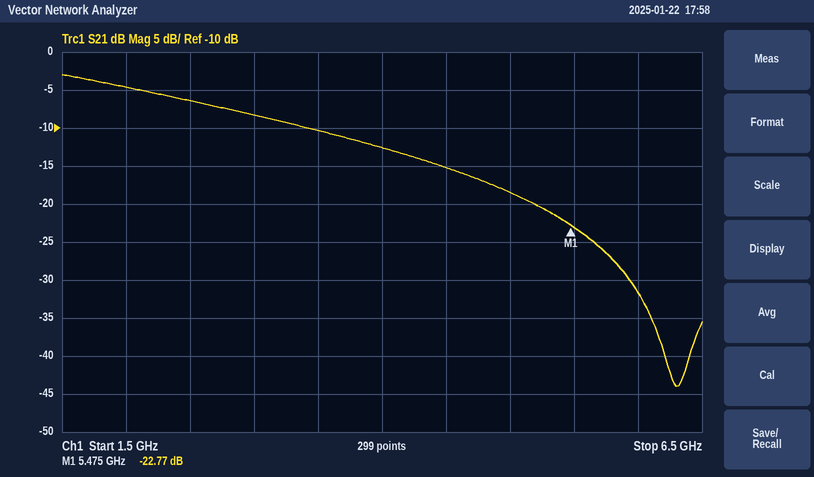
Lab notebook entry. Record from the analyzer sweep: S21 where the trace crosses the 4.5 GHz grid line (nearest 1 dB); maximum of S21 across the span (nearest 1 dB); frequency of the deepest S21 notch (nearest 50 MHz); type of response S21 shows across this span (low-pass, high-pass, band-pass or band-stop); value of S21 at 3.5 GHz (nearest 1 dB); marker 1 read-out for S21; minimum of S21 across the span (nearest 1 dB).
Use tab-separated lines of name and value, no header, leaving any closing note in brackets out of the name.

S21 where the trace crosses the 4.5 GHz grid line	-15 dB
maximum of S21 across the span	-3 dB
frequency of the deepest S21 notch	6.30 GHz
type of response S21 shows across this span	low-pass
value of S21 at 3.5 GHz	-10 dB
marker 1 read-out for S21	-22.77 dB
minimum of S21 across the span	-44 dB
